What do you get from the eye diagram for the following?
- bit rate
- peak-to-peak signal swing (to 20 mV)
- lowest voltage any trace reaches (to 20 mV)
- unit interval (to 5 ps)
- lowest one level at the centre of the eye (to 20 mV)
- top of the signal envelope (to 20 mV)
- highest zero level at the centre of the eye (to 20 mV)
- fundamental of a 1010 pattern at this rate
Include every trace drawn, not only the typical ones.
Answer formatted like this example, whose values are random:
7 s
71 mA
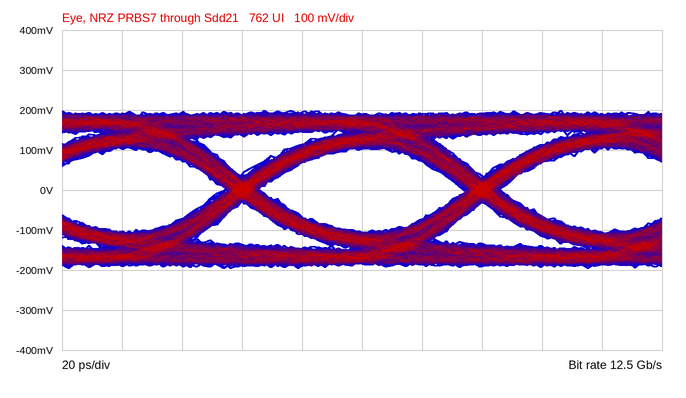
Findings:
12.5 Gb/s
400 mV
-200 mV
80 ps
100 mV
200 mV
-100 mV
6.25 GHz
